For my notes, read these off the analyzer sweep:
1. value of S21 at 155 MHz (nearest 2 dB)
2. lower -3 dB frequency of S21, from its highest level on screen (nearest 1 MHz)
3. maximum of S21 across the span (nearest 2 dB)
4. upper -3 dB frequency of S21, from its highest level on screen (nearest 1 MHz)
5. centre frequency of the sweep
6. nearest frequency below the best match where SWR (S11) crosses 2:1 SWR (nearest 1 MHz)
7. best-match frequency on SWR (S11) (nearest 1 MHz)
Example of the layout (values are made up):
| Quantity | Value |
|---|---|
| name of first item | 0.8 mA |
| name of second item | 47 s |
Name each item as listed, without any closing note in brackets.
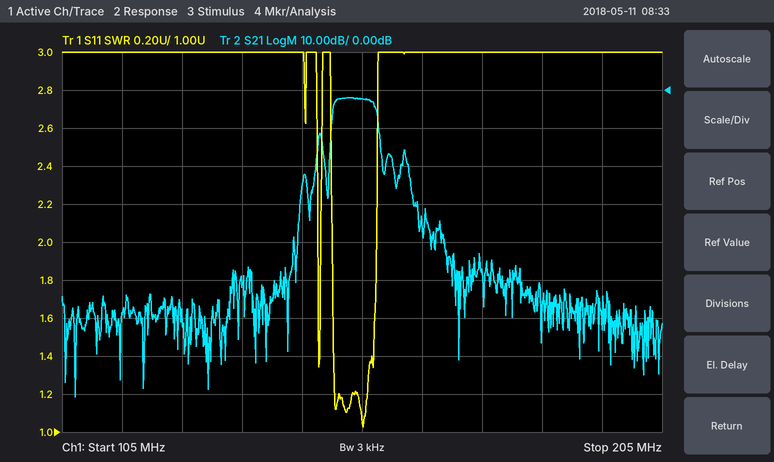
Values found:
| Quantity | Value |
|---|---|
| value of S21 at 155 MHz | -2 dB |
| lower -3 dB frequency of S21, from its highest level on screen | 150 MHz |
| maximum of S21 across the span | -2 dB |
| upper -3 dB frequency of S21, from its highest level on screen | 157 MHz |
| centre frequency of the sweep | 155 MHz |
| nearest frequency below the best match where SWR (S11) crosses 2:1 SWR | 150 MHz |
| best-match frequency on SWR (S11) | 155 MHz |
